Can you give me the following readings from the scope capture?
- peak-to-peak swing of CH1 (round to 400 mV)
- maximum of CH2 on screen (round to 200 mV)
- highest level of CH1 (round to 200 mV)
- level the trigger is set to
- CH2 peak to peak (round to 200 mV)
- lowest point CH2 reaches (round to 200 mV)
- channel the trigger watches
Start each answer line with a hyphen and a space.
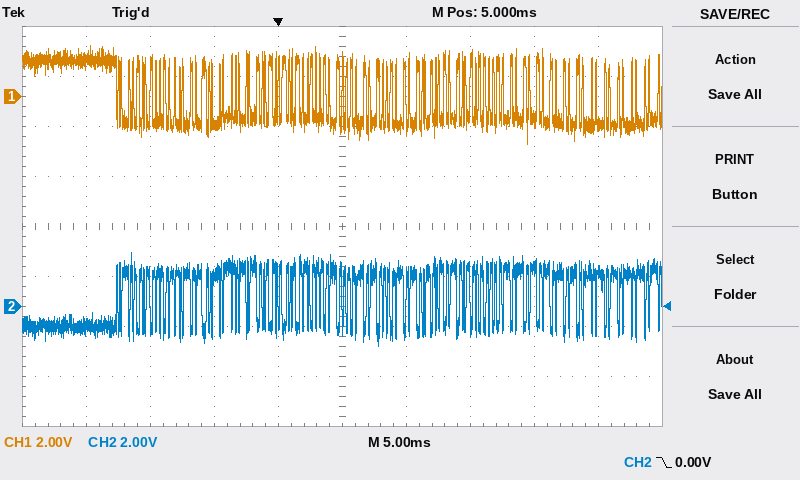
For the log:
- 4.0 V
- 2.2 V
- 2.0 V
- 0.00 V
- 3.8 V
- -1.6 V
- CH2
